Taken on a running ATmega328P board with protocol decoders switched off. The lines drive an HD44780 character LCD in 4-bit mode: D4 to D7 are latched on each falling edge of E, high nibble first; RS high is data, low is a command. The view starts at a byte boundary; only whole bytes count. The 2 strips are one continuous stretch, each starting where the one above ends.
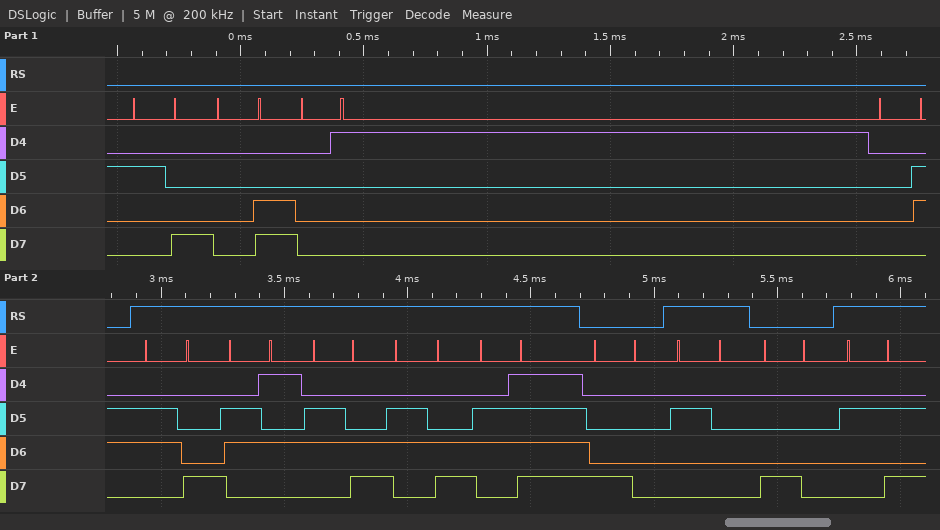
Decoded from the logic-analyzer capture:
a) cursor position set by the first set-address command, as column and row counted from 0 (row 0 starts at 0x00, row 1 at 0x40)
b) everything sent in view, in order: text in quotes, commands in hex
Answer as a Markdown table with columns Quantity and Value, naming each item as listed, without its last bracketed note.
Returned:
| Quantity | Value |
|---|---|
| cursor position set by the first set-address command, as column and row counted from 0 | column 0, row 0 |
| everything sent in view, in order: text in quotes, commands in hex | 0x28 0x0C 0x01 0x06 "hello" 0x80 " " 0x80 "*" |
